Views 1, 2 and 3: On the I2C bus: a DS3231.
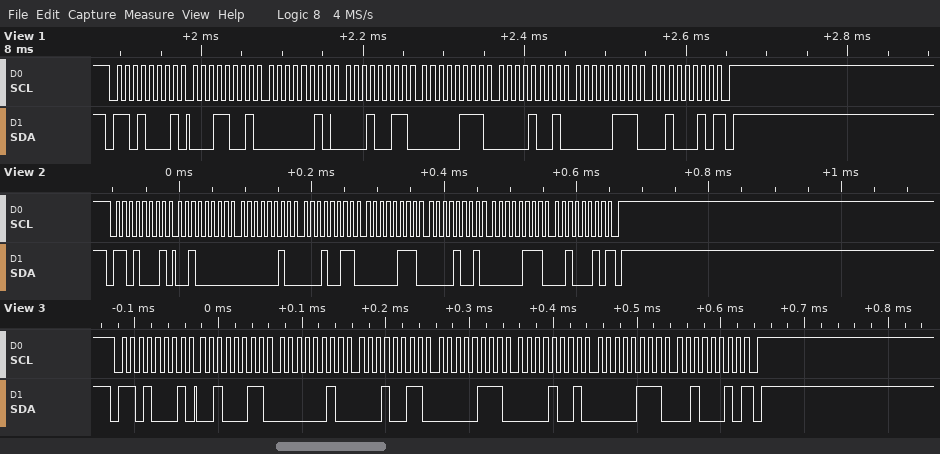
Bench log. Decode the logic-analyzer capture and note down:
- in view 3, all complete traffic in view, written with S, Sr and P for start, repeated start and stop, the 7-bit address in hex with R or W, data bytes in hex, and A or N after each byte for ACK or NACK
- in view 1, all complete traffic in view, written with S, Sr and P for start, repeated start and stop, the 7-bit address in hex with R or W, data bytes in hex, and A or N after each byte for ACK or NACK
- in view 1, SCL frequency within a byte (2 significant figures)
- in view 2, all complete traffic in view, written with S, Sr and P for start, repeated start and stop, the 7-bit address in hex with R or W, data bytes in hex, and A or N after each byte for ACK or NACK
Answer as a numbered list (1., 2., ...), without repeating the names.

1. S 68R A 23 A 02 A 13 A 07 A 09 A 07 A 22 N P
2. S 68R A 19 A 02 A 13 A 07 A 09 A 07 A 22 N P
3. 100 kHz
4. S 68R A 20 A 02 A 13 A 07 A 09 A 07 A 22 N P
